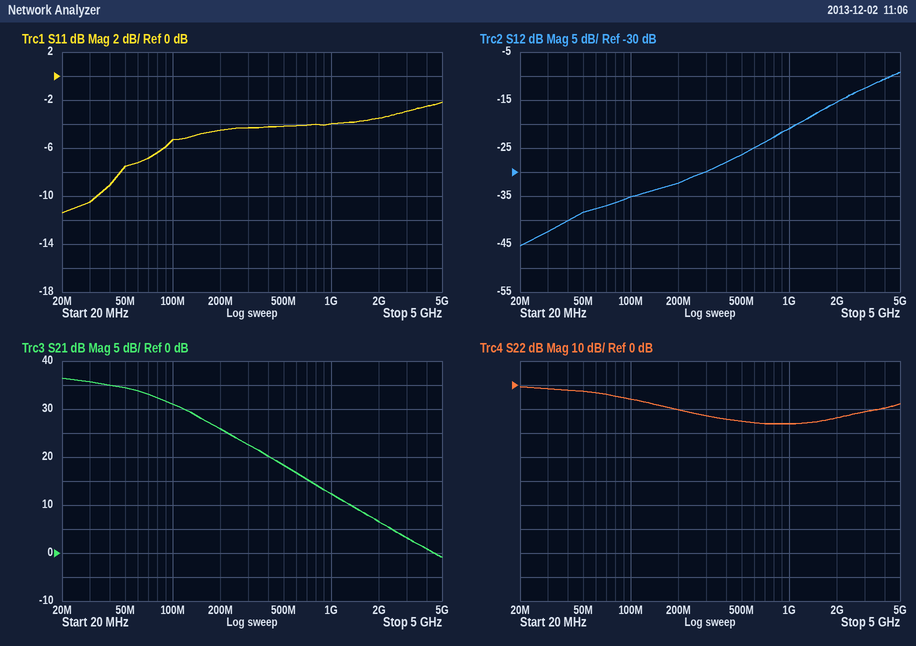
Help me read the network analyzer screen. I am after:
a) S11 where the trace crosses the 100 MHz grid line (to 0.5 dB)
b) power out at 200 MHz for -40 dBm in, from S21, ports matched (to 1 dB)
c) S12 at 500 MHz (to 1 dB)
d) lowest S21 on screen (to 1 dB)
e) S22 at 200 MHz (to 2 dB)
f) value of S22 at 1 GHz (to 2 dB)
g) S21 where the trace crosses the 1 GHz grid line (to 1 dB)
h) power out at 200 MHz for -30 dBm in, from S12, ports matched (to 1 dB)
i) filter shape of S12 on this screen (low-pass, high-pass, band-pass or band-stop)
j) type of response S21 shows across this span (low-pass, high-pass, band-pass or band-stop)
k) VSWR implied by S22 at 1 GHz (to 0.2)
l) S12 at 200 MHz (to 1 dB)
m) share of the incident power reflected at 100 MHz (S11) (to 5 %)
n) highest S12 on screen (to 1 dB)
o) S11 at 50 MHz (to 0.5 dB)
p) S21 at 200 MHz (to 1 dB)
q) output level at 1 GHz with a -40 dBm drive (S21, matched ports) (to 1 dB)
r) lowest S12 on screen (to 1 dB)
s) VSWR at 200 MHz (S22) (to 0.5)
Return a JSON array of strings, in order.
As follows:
["-5.5 dB", "-14 dBm", "-26 dB", "-1 dB", "-10 dB", "-16 dB", "12 dB", "-62 dBm", "high-pass", "low-pass", "1.4", "-32 dB", "30 %", "-9 dB", "-7.5 dB", "26 dB", "-28 dBm", "-45 dB", "2.0"]
